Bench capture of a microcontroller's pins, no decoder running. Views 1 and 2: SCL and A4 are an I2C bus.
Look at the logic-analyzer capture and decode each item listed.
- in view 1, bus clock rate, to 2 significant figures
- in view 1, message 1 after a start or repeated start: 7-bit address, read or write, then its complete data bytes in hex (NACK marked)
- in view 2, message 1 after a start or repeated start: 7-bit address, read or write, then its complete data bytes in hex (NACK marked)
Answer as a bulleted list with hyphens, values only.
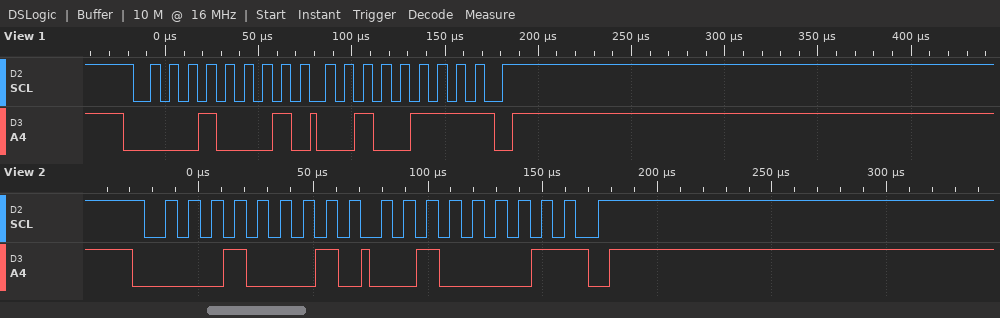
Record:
- 100 kHz
- 0x08 read: 27 NACK
- 0x08 read: 21 NACK
